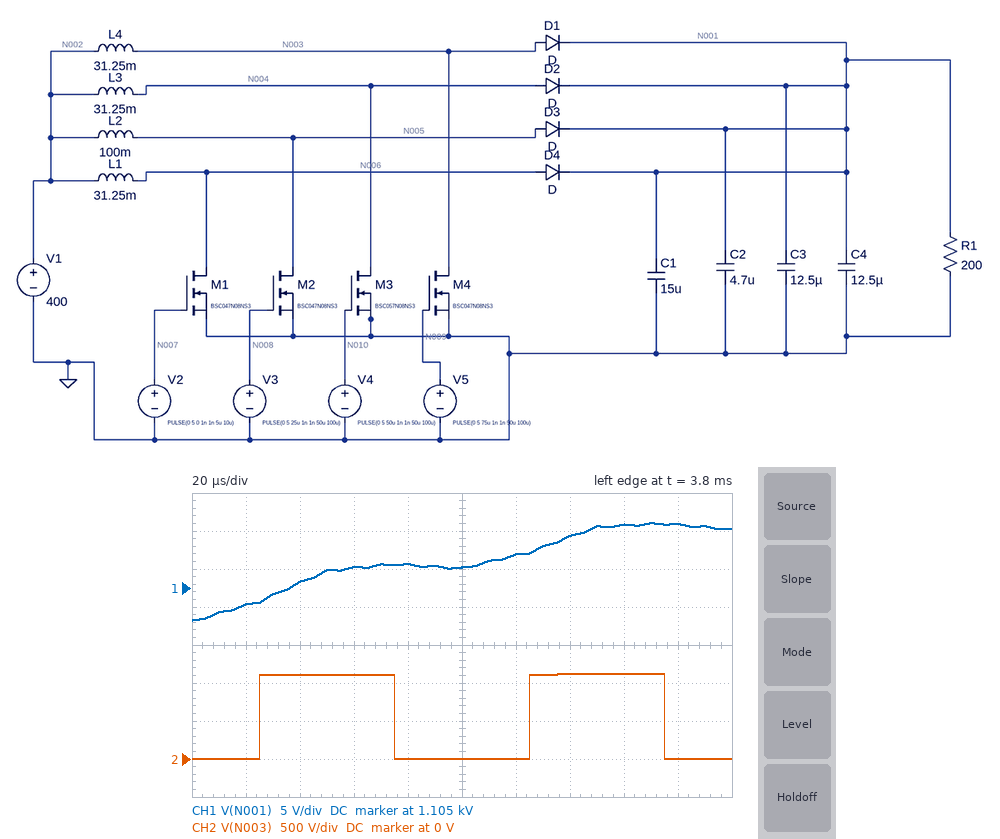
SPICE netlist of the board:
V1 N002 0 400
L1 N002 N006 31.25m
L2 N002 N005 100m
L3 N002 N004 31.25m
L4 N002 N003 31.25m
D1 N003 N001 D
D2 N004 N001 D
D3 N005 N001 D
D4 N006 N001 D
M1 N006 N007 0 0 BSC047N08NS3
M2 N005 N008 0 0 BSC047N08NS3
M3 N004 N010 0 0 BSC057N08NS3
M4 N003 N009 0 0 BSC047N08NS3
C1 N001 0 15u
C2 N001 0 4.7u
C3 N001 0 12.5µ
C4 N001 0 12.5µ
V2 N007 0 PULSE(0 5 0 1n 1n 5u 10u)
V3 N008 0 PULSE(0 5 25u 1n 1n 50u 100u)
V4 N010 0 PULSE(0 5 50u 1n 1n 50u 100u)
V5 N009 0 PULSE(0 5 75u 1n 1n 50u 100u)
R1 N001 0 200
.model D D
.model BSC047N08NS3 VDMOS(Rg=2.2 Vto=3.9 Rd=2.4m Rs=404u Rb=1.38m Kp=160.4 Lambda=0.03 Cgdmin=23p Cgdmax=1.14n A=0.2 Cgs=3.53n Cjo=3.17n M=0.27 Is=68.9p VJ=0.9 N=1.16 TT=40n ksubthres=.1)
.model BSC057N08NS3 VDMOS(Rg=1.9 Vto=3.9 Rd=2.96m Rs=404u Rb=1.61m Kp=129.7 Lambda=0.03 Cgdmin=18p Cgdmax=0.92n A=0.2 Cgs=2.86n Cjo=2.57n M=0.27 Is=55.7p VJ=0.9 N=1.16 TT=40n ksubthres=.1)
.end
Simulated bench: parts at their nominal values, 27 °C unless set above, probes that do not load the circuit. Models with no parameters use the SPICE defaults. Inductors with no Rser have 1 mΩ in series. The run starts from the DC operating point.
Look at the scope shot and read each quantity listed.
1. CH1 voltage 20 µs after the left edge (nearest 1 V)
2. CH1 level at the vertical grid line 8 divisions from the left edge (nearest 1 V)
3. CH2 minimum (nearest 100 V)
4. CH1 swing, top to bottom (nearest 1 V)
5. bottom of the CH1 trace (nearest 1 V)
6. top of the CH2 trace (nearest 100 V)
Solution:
1.103 kV
1.113 kV
0 V
13 V
1.101 kV
1.1 kV
